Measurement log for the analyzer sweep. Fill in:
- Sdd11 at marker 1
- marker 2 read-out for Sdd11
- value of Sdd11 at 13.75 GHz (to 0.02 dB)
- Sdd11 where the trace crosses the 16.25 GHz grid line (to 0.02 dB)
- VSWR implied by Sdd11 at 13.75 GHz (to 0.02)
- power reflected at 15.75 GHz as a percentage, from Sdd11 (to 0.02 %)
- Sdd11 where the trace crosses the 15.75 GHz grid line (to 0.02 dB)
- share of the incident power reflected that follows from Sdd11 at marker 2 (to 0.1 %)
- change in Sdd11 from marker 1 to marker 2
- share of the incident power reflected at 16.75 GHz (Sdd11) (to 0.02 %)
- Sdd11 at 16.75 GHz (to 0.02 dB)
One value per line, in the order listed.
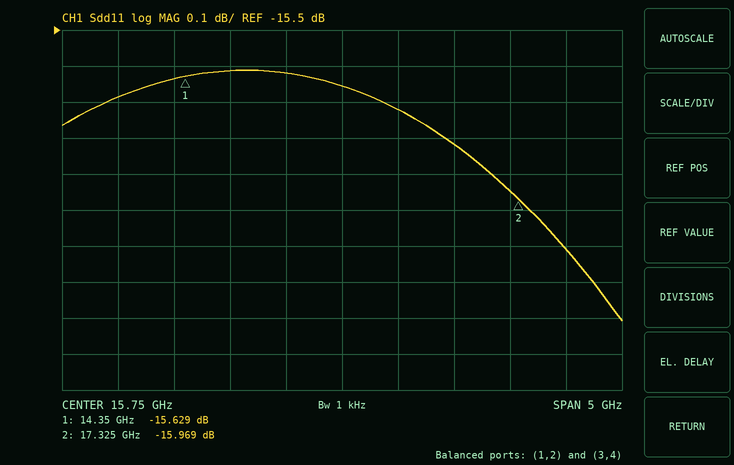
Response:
-15.629 dB
-15.969 dB
-15.68 dB
-15.72 dB
1.40
2.72 %
-15.66 dB
2.5 %
-0.340 dB
2.62 %
-15.82 dB
